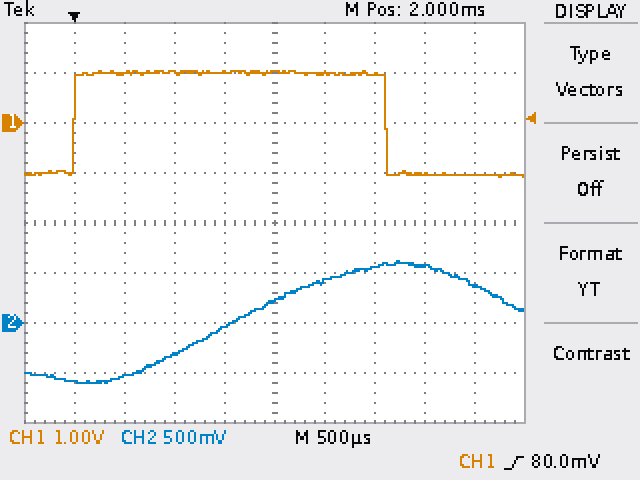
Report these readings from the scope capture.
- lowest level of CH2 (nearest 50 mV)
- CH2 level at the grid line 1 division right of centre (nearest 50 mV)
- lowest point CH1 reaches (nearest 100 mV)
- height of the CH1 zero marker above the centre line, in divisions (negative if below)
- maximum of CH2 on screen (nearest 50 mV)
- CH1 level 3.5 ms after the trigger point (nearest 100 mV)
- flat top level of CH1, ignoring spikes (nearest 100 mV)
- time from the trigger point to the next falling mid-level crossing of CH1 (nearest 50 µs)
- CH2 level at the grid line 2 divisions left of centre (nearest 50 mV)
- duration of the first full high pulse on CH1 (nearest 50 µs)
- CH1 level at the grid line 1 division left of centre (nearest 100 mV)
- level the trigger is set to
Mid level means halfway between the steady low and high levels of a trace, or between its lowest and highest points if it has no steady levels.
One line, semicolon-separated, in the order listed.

-600 mV; 400 mV; -1.1 V; +2.0 div; 600 mV; -1.0 V; 1.0 V; 3.10 ms; -300 mV; 3.10 ms; 1.0 V; 80.0 mV
